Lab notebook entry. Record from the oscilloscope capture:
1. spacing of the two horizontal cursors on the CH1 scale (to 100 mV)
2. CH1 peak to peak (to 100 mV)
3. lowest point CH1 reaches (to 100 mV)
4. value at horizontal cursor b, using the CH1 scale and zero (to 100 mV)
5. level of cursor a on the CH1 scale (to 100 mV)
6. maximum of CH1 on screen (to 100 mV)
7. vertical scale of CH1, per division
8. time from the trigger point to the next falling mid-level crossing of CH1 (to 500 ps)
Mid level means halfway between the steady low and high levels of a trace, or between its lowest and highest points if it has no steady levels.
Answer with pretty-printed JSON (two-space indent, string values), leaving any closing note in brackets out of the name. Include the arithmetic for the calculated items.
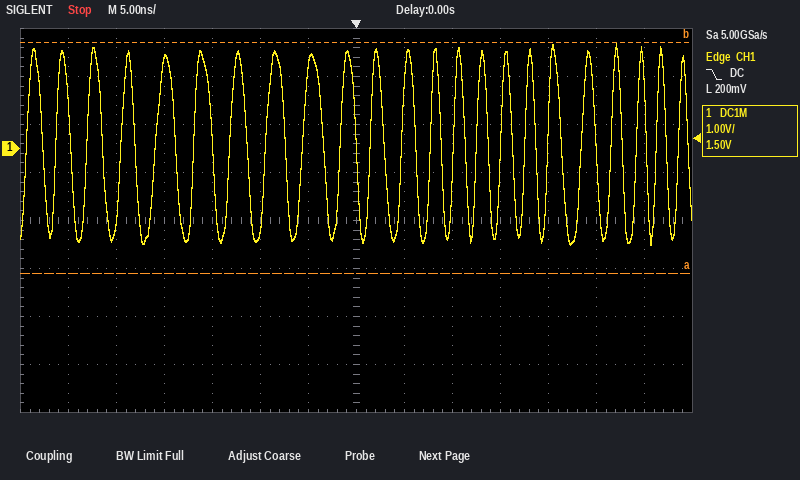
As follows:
{
  "spacing of the two horizontal cursors on the CH1 scale": "4.8 V",
  "CH1 peak to peak": "2.2 V − (-2.0 V) = 4.2 V",
  "lowest point CH1 reaches": "-2.0 V",
  "value at horizontal cursor b, using the CH1 scale and zero": "2.2 V",
  "level of cursor a on the CH1 scale": "-2.6 V",
  "maximum of CH1 on screen": "2.2 V",
  "vertical scale of CH1, per division": "1 V",
  "time from the trigger point to the next falling mid-level crossing of CH1": "3.0 ns"
}
